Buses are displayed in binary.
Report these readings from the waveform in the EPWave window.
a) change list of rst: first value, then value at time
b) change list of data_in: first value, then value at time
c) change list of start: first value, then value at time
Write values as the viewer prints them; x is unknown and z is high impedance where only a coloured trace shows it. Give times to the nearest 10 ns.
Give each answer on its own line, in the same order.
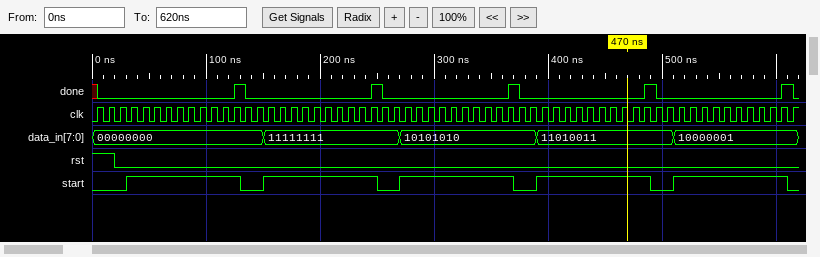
1, 0 at 20 ns
00000000, 11111111 at 150 ns, 10101010 at 270 ns, 11010011 at 390 ns, 10000001 at 510 ns
0, 1 at 30 ns, 0 at 130 ns, 1 at 150 ns, 0 at 250 ns, 1 at 270 ns, 0 at 370 ns, 1 at 390 ns, 0 at 490 ns, 1 at 510 ns, 0 at 610 ns
